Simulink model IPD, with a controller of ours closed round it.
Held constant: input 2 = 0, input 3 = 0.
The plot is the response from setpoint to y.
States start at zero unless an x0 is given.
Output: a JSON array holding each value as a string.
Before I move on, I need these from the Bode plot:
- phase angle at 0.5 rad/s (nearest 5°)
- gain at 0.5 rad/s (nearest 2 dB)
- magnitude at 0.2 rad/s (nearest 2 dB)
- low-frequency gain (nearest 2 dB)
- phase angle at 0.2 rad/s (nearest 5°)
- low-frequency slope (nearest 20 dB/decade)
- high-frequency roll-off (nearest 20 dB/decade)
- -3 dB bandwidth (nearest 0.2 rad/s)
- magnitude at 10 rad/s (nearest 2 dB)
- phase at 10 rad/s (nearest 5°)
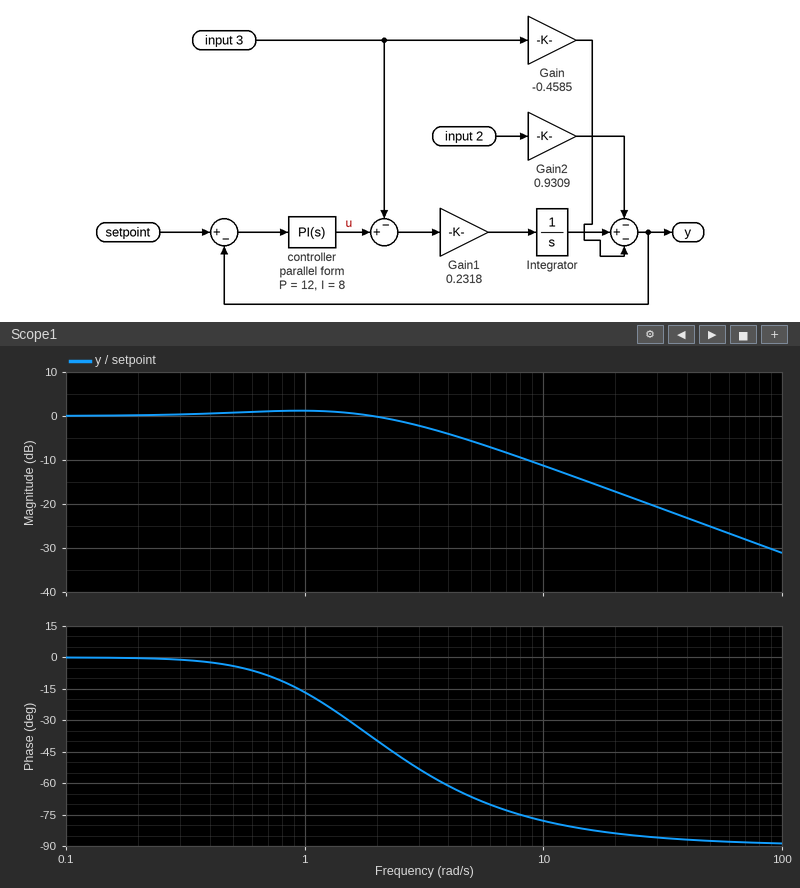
["-5°", "0 dB", "0 dB", "0 dB", "0°", "0 dB/decade", "-20 dB/decade", "3.4 rad/s", "-12 dB", "-80°"]
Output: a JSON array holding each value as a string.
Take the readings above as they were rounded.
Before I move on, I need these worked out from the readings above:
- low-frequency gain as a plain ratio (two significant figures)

["1.0"]
